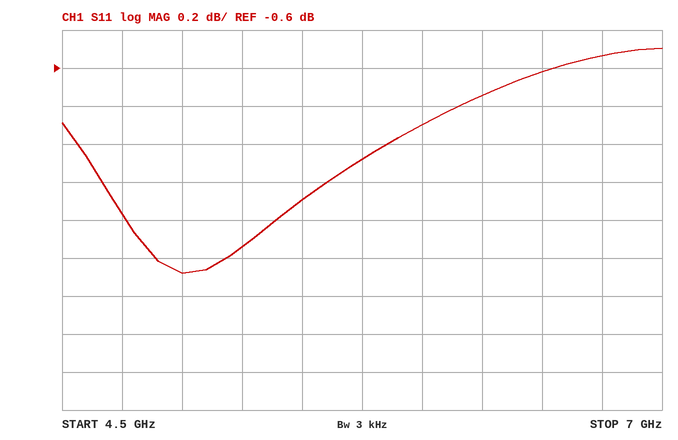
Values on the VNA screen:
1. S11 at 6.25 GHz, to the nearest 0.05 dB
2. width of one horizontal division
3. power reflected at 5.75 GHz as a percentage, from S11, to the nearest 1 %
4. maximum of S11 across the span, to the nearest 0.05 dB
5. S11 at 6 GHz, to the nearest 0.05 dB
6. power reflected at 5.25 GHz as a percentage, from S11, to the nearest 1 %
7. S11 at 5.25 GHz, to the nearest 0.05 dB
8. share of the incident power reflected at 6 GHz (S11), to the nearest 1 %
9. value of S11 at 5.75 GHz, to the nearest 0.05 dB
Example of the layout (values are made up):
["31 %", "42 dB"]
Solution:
["-0.75 dB", "250 MHz", "78 %", "-0.50 dB", "-0.90 dB", "70 %", "-1.55 dB", "81 %", "-1.10 dB"]
